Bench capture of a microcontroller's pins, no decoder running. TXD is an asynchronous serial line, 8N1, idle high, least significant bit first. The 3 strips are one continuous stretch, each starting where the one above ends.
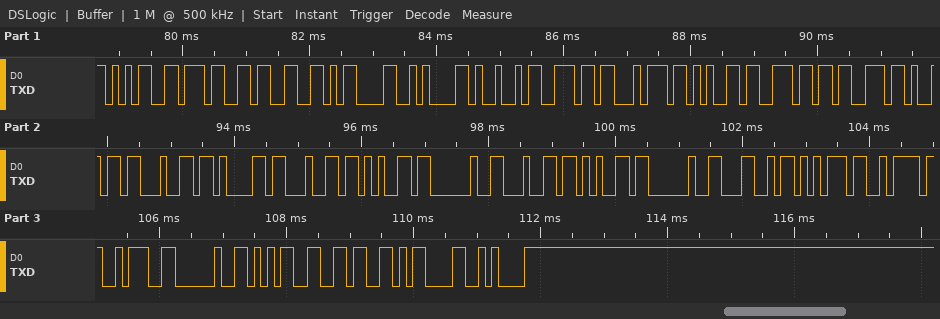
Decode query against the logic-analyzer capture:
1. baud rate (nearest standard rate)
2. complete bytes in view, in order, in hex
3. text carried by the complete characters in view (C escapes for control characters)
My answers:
9600 baud
35 37 33 0D 0A 49 6E 74 65 6E 73 69 64 61 64 65 20 64 65 20 4C 75 7A 3A 20 35 36 0D 0A
"573\r\nIntensidade de Luz: 56\r\n"
